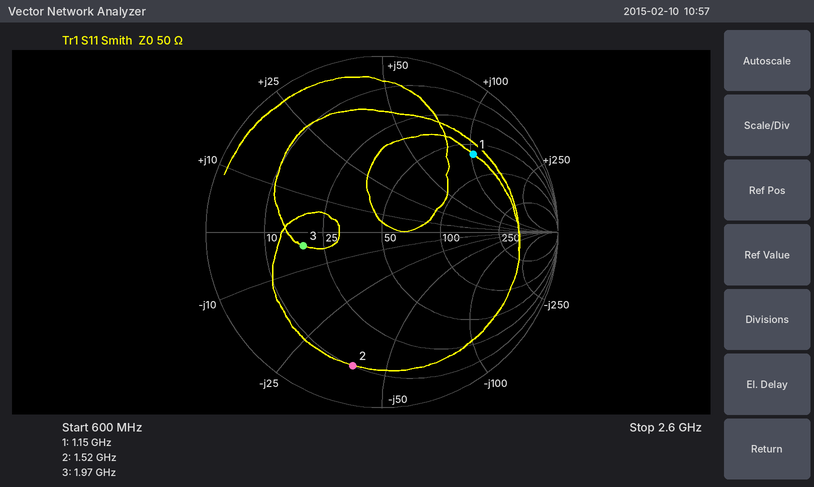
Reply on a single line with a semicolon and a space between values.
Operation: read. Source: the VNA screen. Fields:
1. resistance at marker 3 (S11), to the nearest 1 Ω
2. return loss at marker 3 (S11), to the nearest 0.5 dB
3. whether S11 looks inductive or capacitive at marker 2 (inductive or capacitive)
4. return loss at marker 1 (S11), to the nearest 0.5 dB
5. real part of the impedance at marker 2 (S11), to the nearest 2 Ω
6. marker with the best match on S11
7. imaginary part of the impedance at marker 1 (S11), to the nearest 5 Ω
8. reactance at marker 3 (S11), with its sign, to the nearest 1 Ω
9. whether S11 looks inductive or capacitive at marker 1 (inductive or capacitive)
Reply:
19 Ω; 7.0 dB; capacitive; 3.5 dB; 10 Ω; marker 3; +105 Ω; -4 Ω; inductive
